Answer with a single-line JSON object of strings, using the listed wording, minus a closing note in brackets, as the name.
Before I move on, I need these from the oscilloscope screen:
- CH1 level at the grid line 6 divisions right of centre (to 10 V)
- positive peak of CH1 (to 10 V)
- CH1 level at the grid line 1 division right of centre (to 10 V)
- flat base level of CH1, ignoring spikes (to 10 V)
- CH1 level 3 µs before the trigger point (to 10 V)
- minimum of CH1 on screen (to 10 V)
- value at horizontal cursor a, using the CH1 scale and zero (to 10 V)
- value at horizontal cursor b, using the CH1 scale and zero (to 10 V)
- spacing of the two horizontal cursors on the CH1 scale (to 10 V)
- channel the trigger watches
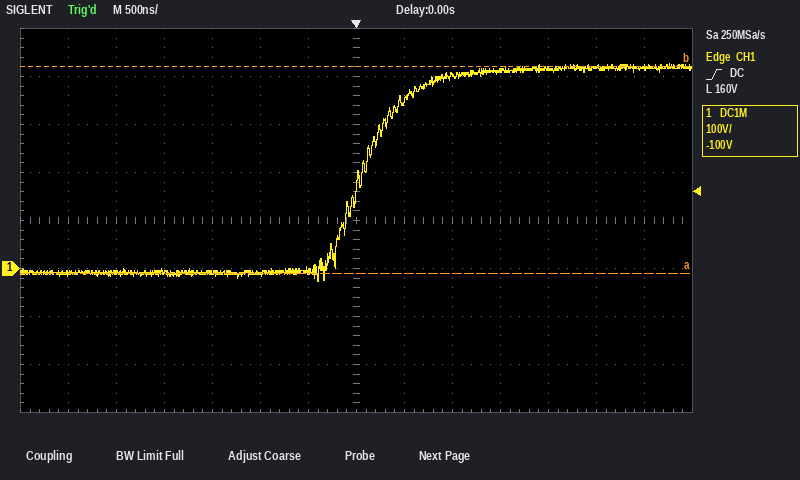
{"CH1 level at the grid line 6 divisions right of centre": "420 V", "positive peak of CH1": "430 V", "CH1 level at the grid line 1 division right of centre": "350 V", "flat base level of CH1, ignoring spikes": "-10 V", "CH1 level 3 µs before the trigger point": "-10 V", "minimum of CH1 on screen": "-30 V", "value at horizontal cursor a, using the CH1 scale and zero": "-10 V", "value at horizontal cursor b, using the CH1 scale and zero": "420 V", "spacing of the two horizontal cursors on the CH1 scale": "430 V", "channel the trigger watches": "CH1"}
